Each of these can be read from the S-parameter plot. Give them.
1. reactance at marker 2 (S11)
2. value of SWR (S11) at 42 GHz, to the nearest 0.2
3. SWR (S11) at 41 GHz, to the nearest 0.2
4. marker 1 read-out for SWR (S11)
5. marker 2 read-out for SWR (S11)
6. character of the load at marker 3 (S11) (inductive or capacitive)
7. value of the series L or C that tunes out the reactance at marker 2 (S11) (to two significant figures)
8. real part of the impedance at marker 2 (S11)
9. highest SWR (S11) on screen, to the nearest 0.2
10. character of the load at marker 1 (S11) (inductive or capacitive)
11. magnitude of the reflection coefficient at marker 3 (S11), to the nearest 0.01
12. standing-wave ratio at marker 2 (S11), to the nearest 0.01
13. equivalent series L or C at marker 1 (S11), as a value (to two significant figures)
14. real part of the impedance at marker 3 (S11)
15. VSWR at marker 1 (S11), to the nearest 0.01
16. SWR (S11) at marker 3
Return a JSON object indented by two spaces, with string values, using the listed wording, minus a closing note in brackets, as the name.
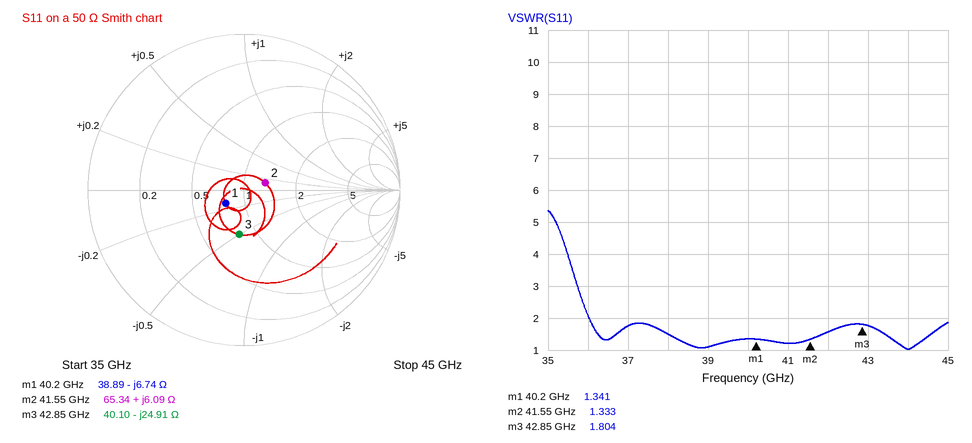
{
  "reactance at marker 2": "+6.09 Ω",
  "value of SWR (S11) at 42 GHz, to the nearest 0.2": "1.6",
  "SWR (S11) at 41 GHz, to the nearest 0.2": "1.2",
  "marker 1 read-out for SWR": "1.341",
  "marker 2 read-out for SWR": "1.333",
  "character of the load at marker 3 (S11)": "capacitive",
  "value of the series L or C that tunes out the reactance at marker 2 (S11)": "630 fF",
  "real part of the impedance at marker 2": "65.34 Ω",
  "highest SWR (S11) on screen, to the nearest 0.2": "5.4",
  "character of the load at marker 1 (S11)": "capacitive",
  "magnitude of the reflection coefficient at marker 3 (S11), to the nearest 0.01": "0.29",
  "standing-wave ratio at marker 2 (S11), to the nearest 0.01": "1.33",
  "equivalent series L or C at marker 1 (S11), as a value": "590 fF",
  "real part of the impedance at marker 3": "40.10 Ω",
  "VSWR at marker 1 (S11), to the nearest 0.01": "1.34",
  "SWR (S11) at marker 3": "1.804"
}
